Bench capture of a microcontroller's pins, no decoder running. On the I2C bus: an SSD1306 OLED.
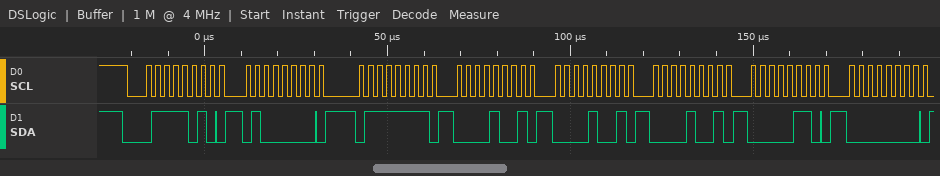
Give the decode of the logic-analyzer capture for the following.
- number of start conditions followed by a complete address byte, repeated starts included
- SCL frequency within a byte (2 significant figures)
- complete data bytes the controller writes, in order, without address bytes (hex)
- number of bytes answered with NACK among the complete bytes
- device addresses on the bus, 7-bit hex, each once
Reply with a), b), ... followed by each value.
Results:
a) 1
b) 400 kHz
c) 40 7F 09 09 09 06 00
d) 0
e) 0x3D
